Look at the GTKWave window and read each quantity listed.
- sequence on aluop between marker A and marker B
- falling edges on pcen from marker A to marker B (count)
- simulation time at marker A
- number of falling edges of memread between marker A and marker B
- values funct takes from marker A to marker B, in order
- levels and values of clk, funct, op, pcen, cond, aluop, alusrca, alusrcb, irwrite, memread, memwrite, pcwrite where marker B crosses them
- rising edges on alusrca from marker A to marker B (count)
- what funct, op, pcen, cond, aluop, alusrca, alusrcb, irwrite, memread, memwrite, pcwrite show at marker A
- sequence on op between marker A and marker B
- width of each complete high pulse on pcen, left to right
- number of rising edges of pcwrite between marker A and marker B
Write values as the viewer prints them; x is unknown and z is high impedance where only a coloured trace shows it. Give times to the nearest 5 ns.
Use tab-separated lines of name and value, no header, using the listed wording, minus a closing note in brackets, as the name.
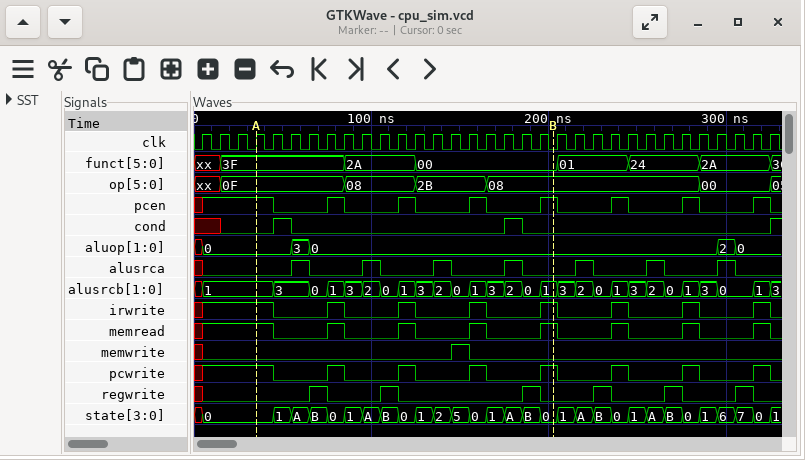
sequence on aluop between marker A and marker B	0, 3, 0
falling edges on pcen from marker A to marker B	4
simulation time at marker A	35 ns
number of falling edges of memread between marker A and marker B	4
values funct takes from marker A to marker B, in order	3F, 2A, 00
levels and values of clk, funct, op, pcen, cond, aluop, alusrca, alusrcb, irwrite, memread, memwrite, pcwrite where marker B crosses them	clk=0, funct=00, op=08, pcen=1, cond=0, aluop=0, alusrca=0, alusrcb=1, irwrite=1, memread=1, memwrite=0, pcwrite=1
rising edges on alusrca from marker A to marker B	4
what funct, op, pcen, cond, aluop, alusrca, alusrcb, irwrite, memread, memwrite, pcwrite show at marker A	funct=3F, op=0F, pcen=1, cond=0, aluop=0, alusrca=0, alusrcb=1, irwrite=1, memread=1, memwrite=0, pcwrite=1
sequence on op between marker A and marker B	0F, 08, 2B, 08
width of each complete high pulse on pcen, left to right	10 ns, 10 ns, 10 ns, 10 ns, 10 ns, 10 ns, 10 ns
number of rising edges of pcwrite between marker A and marker B	4
